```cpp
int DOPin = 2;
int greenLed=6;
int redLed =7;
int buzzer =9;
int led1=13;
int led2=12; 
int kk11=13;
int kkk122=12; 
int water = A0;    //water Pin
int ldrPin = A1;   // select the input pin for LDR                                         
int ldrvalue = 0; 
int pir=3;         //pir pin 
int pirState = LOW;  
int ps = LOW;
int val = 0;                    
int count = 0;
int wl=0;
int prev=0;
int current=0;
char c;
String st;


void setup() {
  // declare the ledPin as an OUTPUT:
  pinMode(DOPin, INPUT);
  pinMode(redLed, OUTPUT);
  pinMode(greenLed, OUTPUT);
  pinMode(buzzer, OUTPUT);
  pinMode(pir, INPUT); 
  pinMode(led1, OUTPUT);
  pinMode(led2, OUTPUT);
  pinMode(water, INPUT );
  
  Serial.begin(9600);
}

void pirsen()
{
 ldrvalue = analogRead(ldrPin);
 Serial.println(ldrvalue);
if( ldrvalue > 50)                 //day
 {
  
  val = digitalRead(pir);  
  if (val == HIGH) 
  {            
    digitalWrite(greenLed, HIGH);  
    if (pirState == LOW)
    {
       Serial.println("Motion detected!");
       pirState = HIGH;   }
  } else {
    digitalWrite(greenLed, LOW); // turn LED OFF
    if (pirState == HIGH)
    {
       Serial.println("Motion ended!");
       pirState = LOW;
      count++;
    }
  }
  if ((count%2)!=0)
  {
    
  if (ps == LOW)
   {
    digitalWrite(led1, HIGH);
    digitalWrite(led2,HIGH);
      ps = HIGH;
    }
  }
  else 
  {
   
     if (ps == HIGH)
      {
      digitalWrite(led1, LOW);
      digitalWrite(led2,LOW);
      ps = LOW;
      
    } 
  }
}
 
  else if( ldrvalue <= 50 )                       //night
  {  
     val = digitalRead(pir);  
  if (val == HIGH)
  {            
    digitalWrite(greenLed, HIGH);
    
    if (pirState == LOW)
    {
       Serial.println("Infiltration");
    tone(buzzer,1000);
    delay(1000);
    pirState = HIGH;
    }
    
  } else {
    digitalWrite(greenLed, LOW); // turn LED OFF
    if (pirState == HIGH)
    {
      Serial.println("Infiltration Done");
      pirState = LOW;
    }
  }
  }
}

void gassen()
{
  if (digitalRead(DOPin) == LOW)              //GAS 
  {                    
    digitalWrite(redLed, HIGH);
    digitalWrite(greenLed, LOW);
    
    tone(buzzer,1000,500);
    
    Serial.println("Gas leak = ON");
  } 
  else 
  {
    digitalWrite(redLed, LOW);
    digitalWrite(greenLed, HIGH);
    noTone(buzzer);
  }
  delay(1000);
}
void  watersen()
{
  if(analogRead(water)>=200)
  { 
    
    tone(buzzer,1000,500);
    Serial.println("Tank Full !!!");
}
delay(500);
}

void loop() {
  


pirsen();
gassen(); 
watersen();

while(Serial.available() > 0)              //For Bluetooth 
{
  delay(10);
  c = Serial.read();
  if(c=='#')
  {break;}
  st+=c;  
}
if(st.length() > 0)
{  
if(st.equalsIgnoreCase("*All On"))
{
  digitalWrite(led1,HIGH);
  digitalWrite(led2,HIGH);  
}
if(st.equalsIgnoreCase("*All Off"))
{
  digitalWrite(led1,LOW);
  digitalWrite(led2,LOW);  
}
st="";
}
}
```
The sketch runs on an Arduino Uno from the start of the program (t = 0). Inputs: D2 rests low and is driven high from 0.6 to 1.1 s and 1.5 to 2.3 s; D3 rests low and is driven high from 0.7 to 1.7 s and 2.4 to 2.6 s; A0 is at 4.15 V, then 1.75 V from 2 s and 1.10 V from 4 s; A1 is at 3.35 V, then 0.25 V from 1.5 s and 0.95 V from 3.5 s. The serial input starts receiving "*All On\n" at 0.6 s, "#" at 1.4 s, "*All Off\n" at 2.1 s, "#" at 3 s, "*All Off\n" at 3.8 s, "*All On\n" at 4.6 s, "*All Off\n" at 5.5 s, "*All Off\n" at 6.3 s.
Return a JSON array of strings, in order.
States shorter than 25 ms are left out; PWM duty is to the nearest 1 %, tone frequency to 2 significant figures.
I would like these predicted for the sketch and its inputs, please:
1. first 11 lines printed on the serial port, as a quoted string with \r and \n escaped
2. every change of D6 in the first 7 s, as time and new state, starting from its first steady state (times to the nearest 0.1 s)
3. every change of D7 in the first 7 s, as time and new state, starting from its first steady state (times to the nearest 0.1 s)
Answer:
["\"686\\r\\nGas leak = ON\\r\\nTank Full !!!\\r\\n51\\r\\nMotion detected!\\r\\nTank Full !!!\\r\\n51\\r\\nMotion ended!\\r\\nGas leak = ON\\r\\nTank Full !!!\\r\\n194\\r\\n\"", "0 s low; 1.6 s high; 3.2 s low", "0 s high; 1.6 s low; 3.2 s high"]
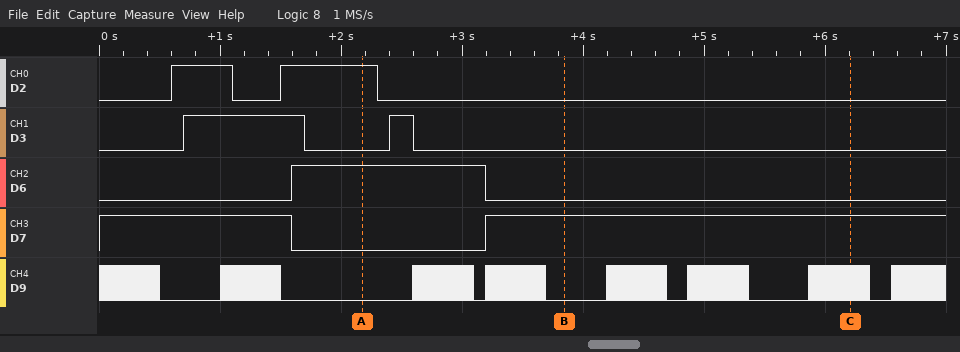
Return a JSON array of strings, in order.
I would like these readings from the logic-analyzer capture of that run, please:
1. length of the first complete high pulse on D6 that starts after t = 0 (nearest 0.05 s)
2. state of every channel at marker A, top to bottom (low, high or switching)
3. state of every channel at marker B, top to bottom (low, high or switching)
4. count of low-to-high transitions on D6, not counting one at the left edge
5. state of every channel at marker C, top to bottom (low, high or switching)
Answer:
["1.60 s", "D2 high, D3 low, D6 high, D7 low, D9 low", "D2 low, D3 low, D6 low, D7 high, D9 low", "1", "D2 low, D3 low, D6 low, D7 high, D9 switching"]
